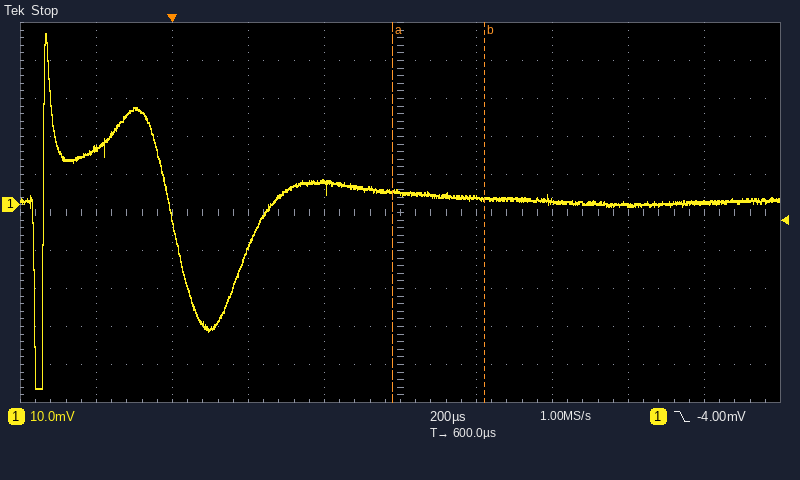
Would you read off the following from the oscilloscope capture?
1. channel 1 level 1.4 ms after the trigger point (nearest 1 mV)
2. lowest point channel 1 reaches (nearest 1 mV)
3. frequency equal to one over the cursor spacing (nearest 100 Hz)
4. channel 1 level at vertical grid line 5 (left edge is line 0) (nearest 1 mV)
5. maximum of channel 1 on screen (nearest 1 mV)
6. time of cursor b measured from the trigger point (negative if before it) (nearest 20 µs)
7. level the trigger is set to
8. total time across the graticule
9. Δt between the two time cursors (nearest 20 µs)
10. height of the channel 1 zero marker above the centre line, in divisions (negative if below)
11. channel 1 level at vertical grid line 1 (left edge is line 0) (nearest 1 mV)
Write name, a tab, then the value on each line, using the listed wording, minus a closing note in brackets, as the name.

channel 1 level 1.4 ms after the trigger point	1 mV
lowest point channel 1 reaches	-48 mV
frequency equal to one over the cursor spacing	4.2 kHz
channel 1 level at vertical grid line 5 (left edge is line 0)	3 mV
maximum of channel 1 on screen	45 mV
time of cursor b measured from the trigger point (negative if before it)	+820 µs
level the trigger is set to	-4.00 mV
total time across the graticule	2 ms
Δt between the two time cursors	240 µs
height of the channel 1 zero marker above the centre line, in divisions	+0.2 div
channel 1 level at vertical grid line 1 (left edge is line 0)	15 mV
